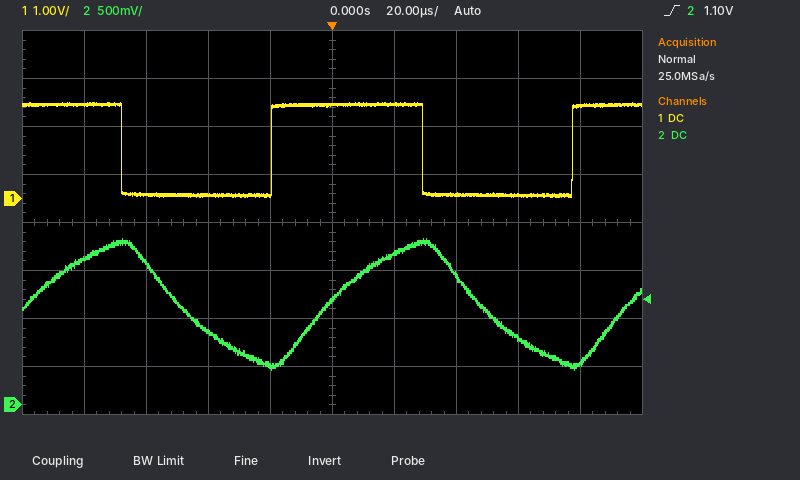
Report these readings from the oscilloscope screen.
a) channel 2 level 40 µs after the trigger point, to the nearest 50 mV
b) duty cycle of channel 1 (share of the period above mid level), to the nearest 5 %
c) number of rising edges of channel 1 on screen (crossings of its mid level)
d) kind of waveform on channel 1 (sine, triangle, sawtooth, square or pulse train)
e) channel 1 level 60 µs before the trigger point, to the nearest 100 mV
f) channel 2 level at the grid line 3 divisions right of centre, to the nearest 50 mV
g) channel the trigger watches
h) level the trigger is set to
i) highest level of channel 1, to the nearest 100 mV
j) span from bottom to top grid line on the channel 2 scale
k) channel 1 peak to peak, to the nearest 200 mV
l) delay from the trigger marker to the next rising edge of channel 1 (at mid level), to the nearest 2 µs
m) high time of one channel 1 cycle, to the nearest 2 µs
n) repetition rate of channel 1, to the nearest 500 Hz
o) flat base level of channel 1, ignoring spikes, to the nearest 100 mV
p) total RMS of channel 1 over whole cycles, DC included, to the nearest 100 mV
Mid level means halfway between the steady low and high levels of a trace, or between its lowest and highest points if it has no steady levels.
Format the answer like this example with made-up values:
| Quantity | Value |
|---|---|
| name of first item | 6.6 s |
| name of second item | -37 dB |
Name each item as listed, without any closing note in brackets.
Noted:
| Quantity | Value |
|---|---|
| channel 2 level 40 µs after the trigger point, to the nearest 50 mV | 1.35 V |
| duty cycle of channel 1 (share of the period above mid level), to the nearest 5 % | 50 % |
| number of rising edges of channel 1 on screen | 2 |
| kind of waveform on channel 1 | square |
| channel 1 level 60 µs before the trigger point, to the nearest 100 mV | 100 mV |
| channel 2 level at the grid line 3 divisions right of centre, to the nearest 50 mV | 700 mV |
| channel the trigger watches | channel 2 |
| level the trigger is set to | 1.10 V |
| highest level of channel 1, to the nearest 100 mV | 2.0 V |
| span from bottom to top grid line on the channel 2 scale | 4 V |
| channel 1 peak to peak, to the nearest 200 mV | 2.0 V |
| delay from the trigger marker to the next rising edge of channel 1 (at mid level), to the nearest 2 µs | 78 µs |
| high time of one channel 1 cycle, to the nearest 2 µs | 48 µs |
| repetition rate of channel 1, to the nearest 500 Hz | 10.5 kHz |
| flat base level of channel 1, ignoring spikes, to the nearest 100 mV | 100 mV |
| total RMS of channel 1 over whole cycles, DC included, to the nearest 100 mV | 1.4 V |
